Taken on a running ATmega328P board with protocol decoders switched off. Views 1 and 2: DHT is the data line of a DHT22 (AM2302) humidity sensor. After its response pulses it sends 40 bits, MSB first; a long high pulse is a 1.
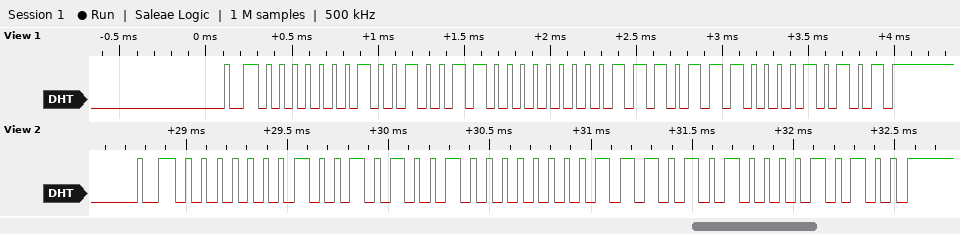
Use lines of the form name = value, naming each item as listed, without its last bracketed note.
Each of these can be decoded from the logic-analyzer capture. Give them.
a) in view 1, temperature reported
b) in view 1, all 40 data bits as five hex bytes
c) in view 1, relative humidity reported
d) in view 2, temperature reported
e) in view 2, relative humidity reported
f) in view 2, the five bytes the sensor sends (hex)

in view 1, temperature reported = 23.8 °C
in view 1, all 40 data bits as five hex bytes = 01 26 00 EE 15
in view 1, relative humidity reported = 29.4 %
in view 2, temperature reported = 23.4 °C
in view 2, relative humidity reported = 29.7 %
in view 2, the five bytes the sensor sends = 01 29 00 EA 14
